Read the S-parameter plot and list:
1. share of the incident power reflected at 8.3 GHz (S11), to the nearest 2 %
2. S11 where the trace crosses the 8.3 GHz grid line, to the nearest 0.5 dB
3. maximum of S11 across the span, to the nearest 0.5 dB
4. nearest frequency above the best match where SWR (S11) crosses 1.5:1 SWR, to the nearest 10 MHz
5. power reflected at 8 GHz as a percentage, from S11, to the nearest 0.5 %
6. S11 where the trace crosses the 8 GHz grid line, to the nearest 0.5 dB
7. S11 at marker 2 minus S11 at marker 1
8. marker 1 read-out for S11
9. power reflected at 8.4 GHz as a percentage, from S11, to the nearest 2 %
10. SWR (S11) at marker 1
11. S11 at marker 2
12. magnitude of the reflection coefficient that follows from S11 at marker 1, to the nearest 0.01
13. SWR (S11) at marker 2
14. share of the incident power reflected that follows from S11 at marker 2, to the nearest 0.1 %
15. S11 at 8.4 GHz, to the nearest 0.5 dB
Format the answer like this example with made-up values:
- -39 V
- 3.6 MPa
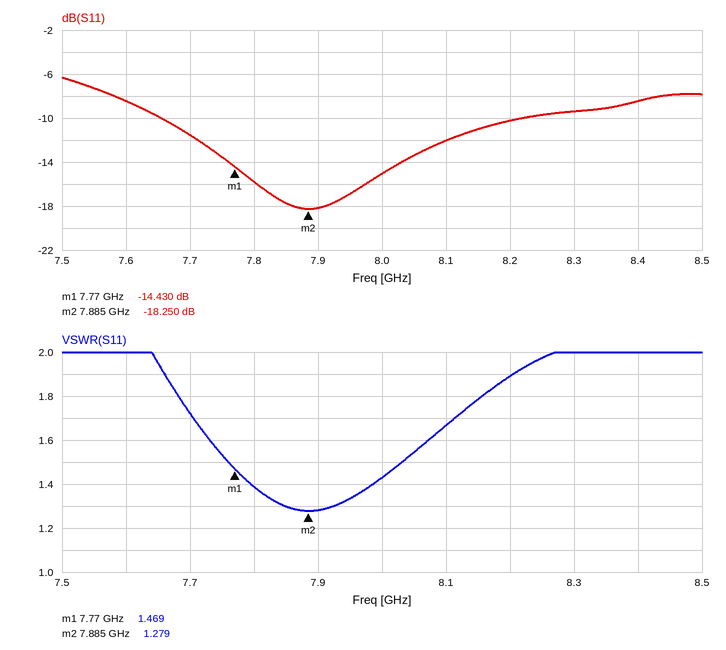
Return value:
- 12 %
- -9.5 dB
- -6.5 dB
- 8.03 GHz
- 3.0 %
- -15.0 dB
- -3.820 dB
- -14.430 dB
- 14 %
- 1.469
- -18.250 dB
- 0.19
- 1.279
- 1.5 %
- -8.5 dB
